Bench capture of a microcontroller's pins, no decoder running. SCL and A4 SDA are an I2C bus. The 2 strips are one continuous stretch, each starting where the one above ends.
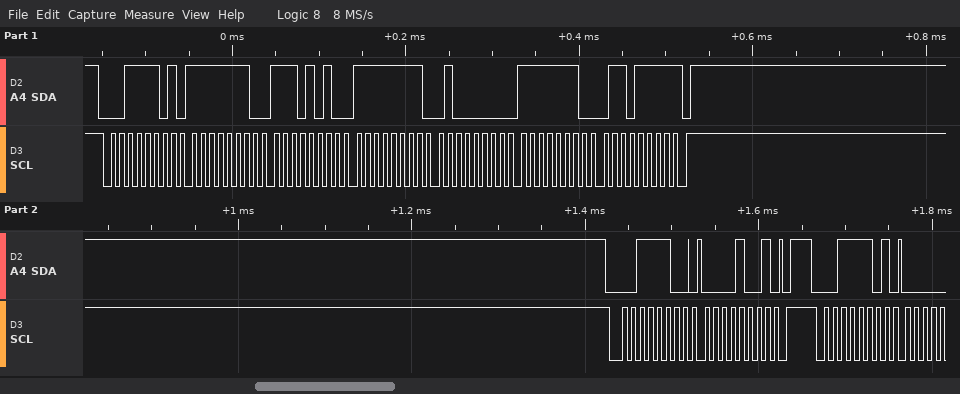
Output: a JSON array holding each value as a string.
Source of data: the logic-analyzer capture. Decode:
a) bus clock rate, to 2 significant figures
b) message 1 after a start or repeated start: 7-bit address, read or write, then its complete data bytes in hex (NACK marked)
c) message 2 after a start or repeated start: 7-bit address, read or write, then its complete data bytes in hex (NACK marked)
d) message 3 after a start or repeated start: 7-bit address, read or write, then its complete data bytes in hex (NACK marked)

["100 kHz", "0x1E read: FE EA FF 40 FE 6F NACK", "0x1E write: 09", "0x1E read"]
